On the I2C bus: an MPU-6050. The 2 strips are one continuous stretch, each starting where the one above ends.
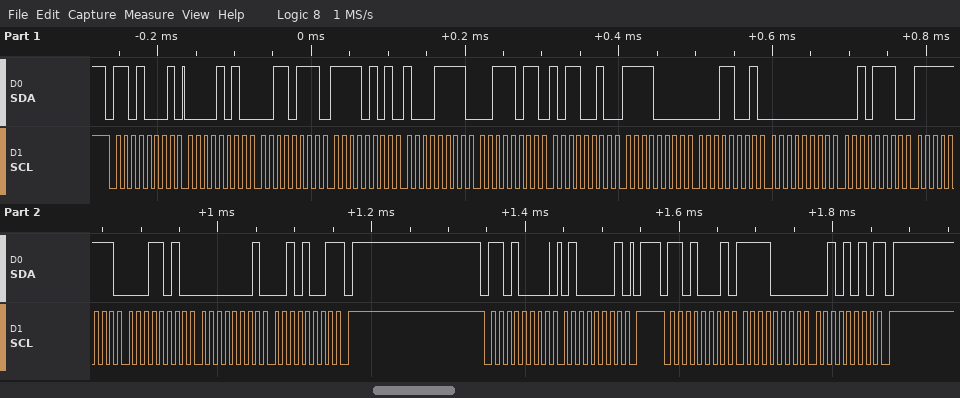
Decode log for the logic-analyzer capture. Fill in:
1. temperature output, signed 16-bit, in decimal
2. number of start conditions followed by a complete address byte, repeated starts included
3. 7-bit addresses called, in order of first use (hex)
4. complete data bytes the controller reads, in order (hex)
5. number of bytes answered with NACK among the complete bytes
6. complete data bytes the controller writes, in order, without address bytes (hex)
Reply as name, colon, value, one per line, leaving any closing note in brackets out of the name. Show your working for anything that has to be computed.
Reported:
temperature output, signed 16-bit, in decimal: 0xF02A = -4054
number of start conditions followed by a complete address byte, repeated starts included: 3
7-bit addresses called, in order of first use: 0x68
complete data bytes the controller reads, in order: 0A 37 F5 8F 3B B2 F0 19 00 2E FF 1A 01 29 F0 2A
number of bytes answered with NACK among the complete bytes: 2
complete data bytes the controller writes, in order, without address bytes: 41
